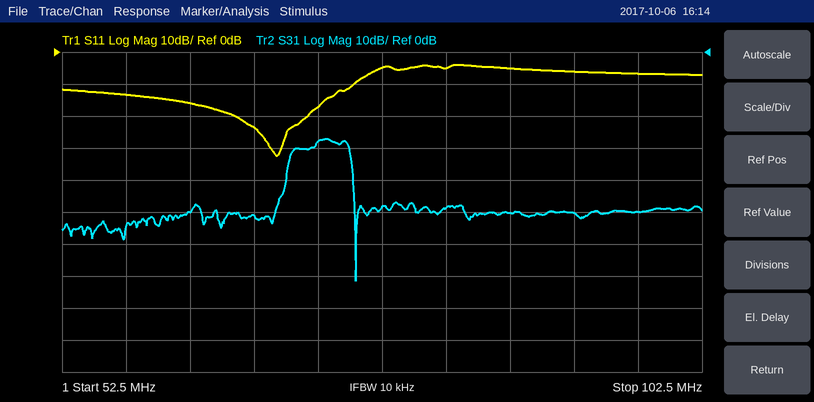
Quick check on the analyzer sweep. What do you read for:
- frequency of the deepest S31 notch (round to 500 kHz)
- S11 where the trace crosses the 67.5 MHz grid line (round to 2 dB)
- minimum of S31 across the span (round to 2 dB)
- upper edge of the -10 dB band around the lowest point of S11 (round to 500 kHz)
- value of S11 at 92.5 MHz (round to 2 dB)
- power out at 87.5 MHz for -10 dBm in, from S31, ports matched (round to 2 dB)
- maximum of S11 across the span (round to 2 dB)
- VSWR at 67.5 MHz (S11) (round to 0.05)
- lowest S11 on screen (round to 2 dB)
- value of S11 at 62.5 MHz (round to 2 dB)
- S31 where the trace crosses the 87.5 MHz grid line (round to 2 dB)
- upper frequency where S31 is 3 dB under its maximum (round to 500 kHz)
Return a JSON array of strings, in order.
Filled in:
["75.5 MHz", "-24 dB", "-72 dB", "75.5 MHz", "-6 dB", "-60 dBm", "-4 dB", "1.15", "-32 dB", "-16 dB", "-50 dB", "75.0 MHz"]
